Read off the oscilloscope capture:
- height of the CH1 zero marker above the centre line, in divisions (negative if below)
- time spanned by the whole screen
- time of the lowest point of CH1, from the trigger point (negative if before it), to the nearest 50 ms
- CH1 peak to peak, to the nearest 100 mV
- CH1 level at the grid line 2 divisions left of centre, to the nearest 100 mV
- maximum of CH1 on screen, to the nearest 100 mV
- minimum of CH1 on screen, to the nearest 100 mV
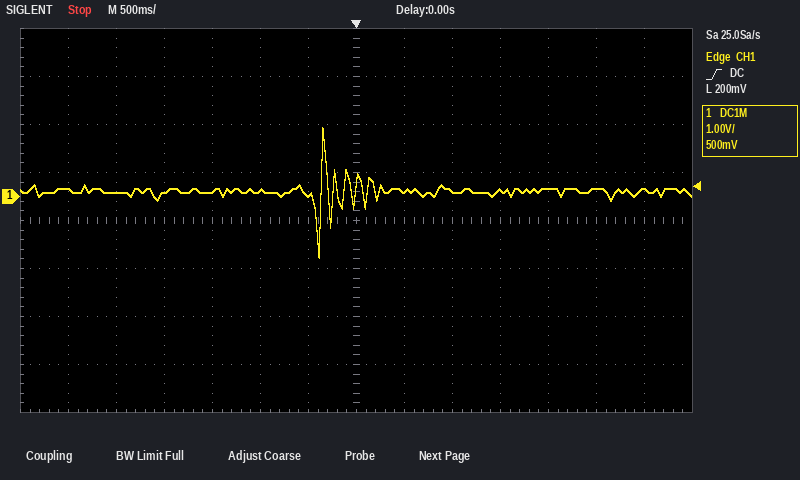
+0.5 div
7 s
-400 ms
2.7 V
100 mV
1.4 V
-1.3 V
